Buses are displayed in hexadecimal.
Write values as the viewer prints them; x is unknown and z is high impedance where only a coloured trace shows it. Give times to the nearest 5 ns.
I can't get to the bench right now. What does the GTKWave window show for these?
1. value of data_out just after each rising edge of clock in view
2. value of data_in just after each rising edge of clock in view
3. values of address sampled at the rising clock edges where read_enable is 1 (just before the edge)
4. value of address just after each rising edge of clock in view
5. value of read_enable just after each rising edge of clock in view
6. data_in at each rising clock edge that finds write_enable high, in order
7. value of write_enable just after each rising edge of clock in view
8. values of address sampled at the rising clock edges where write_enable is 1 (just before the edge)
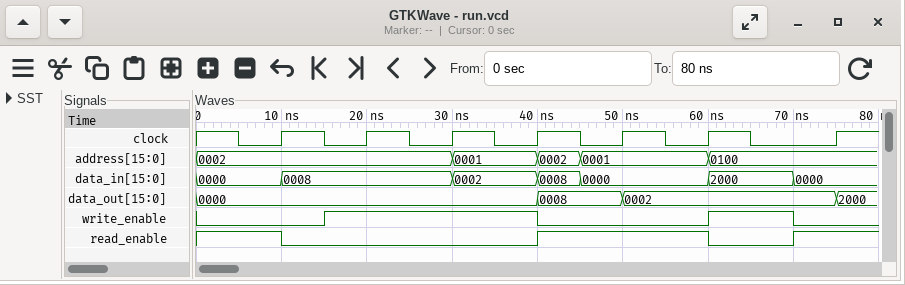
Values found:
0000, 0000, 0000, 0008, 0002, 0002, 2000
0008, 0008, 0002, 0008, 0000, 2000, 0000
0002, 0001, 0001, 0100
0002, 0002, 0001, 0002, 0001, 0100, 0100
0 0 0 1 1 0 1
0008, 0008, 0002
0 1 1 0 0 1 0
0002, 0002, 0001
